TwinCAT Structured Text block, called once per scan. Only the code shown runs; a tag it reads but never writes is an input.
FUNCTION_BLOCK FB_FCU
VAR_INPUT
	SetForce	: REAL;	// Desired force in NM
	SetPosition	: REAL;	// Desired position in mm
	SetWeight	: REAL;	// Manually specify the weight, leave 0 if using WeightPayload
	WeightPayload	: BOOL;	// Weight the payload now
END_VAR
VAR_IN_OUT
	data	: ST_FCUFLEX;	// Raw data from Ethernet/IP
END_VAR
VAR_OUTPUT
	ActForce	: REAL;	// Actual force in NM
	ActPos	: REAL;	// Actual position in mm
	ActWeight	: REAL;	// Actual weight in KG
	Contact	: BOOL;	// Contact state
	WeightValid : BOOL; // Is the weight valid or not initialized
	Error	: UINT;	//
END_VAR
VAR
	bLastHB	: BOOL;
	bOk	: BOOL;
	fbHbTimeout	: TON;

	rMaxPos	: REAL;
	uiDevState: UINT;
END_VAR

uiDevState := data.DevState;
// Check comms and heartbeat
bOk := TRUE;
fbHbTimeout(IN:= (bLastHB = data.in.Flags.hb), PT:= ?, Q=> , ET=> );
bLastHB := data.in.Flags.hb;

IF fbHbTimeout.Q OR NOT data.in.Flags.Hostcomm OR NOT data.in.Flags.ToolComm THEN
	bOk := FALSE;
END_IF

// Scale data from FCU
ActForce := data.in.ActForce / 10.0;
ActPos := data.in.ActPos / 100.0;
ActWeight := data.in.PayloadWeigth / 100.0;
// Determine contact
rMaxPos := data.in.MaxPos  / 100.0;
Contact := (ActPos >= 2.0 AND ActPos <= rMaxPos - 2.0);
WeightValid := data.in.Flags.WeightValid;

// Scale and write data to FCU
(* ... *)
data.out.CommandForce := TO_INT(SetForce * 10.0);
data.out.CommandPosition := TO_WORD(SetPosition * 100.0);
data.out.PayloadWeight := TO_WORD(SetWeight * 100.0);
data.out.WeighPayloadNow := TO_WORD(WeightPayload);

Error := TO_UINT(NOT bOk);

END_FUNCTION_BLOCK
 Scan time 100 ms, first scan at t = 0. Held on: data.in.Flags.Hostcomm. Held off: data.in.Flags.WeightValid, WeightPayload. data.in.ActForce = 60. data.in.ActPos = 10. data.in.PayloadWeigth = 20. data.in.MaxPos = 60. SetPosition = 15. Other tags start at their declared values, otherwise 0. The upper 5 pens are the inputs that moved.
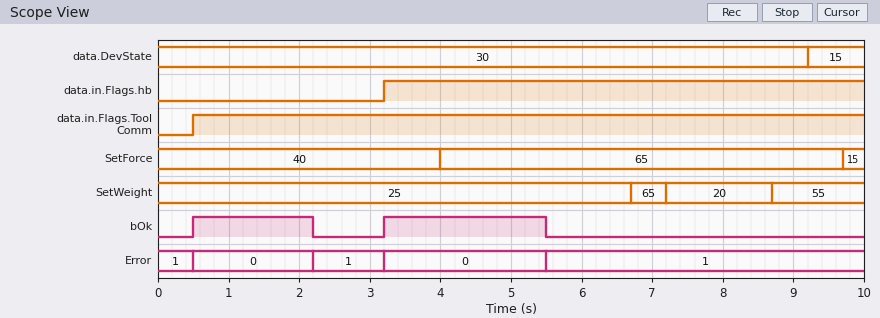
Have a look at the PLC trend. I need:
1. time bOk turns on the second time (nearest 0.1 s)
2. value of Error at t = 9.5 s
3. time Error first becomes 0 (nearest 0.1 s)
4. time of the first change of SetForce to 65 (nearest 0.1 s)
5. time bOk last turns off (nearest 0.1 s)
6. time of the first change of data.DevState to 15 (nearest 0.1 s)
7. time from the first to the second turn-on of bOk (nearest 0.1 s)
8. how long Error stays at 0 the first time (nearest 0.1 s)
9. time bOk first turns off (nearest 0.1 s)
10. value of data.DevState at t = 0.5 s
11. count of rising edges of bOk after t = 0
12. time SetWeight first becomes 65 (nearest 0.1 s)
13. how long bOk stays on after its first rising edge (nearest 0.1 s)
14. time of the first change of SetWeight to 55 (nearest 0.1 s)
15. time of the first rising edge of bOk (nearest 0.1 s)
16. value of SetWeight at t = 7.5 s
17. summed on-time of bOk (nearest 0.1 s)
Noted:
3.2 s
1
0.5 s
4.0 s
5.5 s
9.2 s
2.7 s
1.7 s
2.2 s
30
2
6.7 s
1.7 s
8.7 s
0.5 s
20
4.0 s
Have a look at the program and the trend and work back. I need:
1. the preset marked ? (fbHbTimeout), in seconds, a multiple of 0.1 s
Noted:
2.2 s
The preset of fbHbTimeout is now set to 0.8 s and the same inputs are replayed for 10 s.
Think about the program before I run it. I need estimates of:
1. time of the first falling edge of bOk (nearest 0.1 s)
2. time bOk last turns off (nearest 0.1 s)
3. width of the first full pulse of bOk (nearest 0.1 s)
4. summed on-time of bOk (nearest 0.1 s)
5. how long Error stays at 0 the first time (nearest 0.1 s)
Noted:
0.8 s
4.1 s
0.3 s
1.2 s
0.3 s
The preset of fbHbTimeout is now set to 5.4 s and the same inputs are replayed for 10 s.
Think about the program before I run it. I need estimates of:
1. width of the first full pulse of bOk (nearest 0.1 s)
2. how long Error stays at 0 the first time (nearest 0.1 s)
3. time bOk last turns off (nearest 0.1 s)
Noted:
8.2 s
8.2 s
8.7 s
